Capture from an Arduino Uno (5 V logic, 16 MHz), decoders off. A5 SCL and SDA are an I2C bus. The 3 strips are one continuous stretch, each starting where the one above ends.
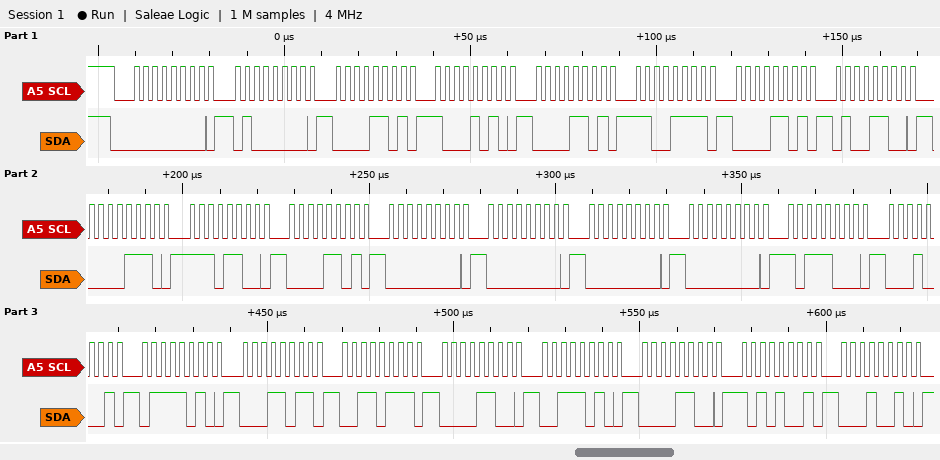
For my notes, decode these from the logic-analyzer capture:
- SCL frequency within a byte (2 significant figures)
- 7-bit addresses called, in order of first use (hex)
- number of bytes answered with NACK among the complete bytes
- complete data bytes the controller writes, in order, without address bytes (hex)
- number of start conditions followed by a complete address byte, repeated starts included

400 kHz
0x00
0
40 0D 8A 0D CF 0D 4C 0E EC 0D 00 00 00 00 B8 11 7A 1B 37 0C 3A 0C A9 12
1
